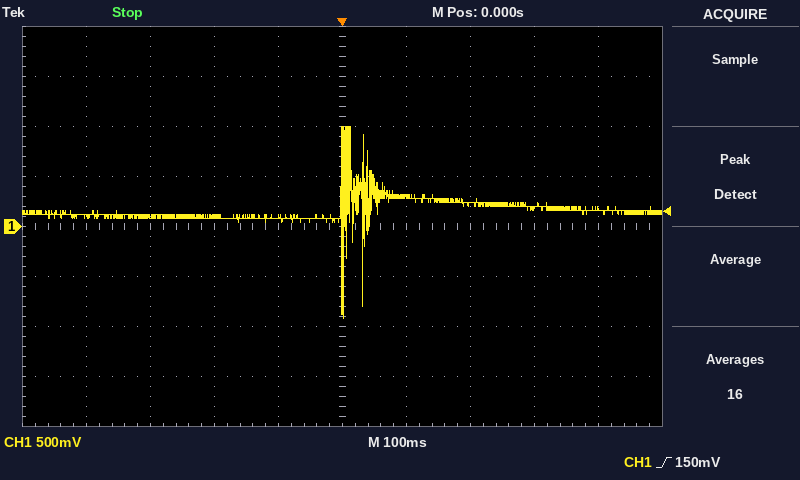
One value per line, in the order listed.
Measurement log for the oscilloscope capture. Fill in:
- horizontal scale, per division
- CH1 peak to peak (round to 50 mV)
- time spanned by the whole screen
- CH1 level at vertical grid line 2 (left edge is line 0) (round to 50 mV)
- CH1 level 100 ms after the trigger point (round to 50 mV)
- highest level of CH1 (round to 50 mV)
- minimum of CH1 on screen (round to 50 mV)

100 ms
1.90 V
1 s
100 mV
300 mV
1.00 V
-900 mV
